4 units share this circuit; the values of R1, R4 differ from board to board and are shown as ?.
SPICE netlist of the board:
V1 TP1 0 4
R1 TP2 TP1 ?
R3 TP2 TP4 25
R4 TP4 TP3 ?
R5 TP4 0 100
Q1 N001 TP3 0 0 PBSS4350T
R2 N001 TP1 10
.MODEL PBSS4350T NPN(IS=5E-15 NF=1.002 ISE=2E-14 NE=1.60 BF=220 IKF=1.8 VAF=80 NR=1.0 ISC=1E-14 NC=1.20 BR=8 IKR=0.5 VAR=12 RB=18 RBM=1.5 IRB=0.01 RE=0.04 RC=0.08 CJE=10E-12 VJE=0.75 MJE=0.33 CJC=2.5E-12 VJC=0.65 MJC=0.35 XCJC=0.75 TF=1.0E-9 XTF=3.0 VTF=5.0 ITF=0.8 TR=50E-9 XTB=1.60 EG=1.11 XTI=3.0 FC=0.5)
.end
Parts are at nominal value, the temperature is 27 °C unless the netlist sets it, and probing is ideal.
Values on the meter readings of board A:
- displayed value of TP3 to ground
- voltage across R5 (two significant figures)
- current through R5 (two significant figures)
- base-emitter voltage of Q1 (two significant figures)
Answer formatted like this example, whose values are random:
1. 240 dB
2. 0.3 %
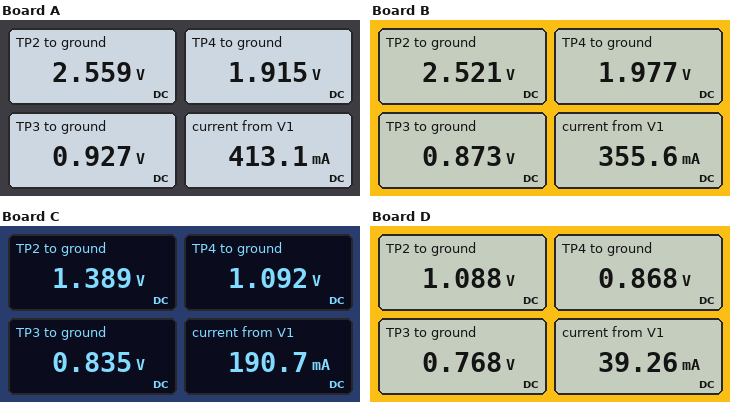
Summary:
1. 0.927 V
2. 1.9 V
3. 19 mA
4. 930 mV
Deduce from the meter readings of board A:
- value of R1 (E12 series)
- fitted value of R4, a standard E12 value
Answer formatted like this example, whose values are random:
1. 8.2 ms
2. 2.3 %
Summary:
1. 56 Ω
2. 150 Ω
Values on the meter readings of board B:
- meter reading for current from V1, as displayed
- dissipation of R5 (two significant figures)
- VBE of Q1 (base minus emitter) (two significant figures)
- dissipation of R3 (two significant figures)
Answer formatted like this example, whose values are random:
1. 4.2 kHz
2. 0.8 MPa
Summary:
1. 355.6 mA
2. 39 mW
3. 870 mV
4. 12 mW
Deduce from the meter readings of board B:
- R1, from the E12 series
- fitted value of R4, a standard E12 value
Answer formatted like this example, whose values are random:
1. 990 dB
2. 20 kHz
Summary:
1. 68 Ω
2. 560 Ω
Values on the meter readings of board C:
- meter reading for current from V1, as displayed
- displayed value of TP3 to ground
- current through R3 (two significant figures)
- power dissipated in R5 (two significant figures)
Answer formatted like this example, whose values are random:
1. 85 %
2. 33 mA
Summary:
1. 190.7 mA
2. 0.835 V
3. 12 mA
4. 12 mW
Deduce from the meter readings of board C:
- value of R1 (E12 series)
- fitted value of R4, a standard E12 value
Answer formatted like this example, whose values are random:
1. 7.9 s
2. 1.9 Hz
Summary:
1. 220 Ω
2. 270 Ω
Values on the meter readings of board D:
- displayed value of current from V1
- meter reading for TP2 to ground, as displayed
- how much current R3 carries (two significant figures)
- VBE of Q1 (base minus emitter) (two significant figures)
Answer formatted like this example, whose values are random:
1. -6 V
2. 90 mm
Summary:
1. 39.26 mA
2. 1.088 V
3. 8.8 mA
4. 770 mV
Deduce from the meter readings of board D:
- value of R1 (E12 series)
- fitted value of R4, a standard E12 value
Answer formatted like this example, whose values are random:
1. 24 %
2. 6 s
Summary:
1. 330 Ω
2. 680 Ω
